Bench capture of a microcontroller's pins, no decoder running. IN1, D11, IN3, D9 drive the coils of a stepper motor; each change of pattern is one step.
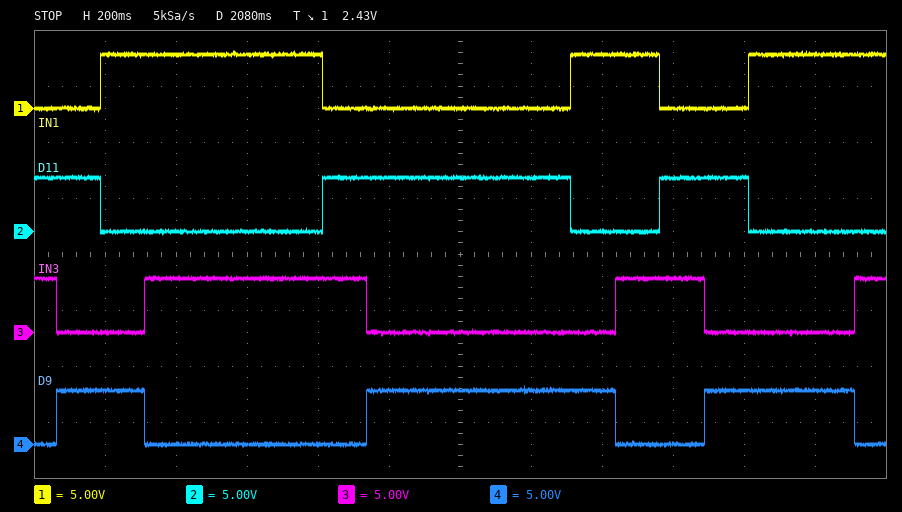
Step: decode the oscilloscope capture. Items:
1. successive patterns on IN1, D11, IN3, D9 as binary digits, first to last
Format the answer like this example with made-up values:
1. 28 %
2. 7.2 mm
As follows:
1. 0110 0101 1001 1010 0110 0101 1001 1010 0110 0101 1001 1010
